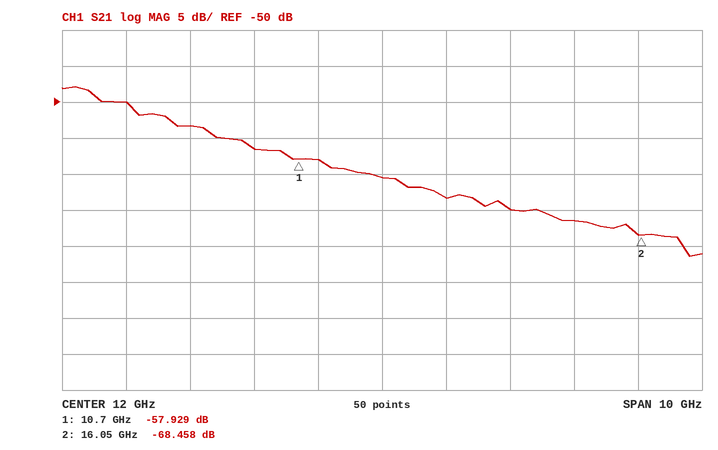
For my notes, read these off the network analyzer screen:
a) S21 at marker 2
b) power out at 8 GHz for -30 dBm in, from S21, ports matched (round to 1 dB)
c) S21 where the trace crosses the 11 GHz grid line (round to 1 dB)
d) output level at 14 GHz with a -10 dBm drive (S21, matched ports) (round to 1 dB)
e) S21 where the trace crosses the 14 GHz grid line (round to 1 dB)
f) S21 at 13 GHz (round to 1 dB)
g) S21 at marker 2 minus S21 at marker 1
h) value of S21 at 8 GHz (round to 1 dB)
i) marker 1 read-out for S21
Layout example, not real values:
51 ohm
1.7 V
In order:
-68.458 dB
-80 dBm
-58 dB
-75 dBm
-65 dB
-63 dB
-10.529 dB
-50 dB
-57.929 dB
